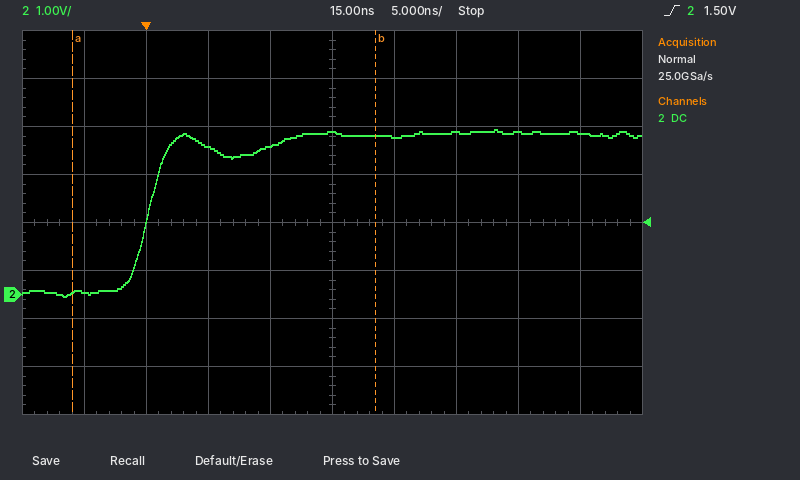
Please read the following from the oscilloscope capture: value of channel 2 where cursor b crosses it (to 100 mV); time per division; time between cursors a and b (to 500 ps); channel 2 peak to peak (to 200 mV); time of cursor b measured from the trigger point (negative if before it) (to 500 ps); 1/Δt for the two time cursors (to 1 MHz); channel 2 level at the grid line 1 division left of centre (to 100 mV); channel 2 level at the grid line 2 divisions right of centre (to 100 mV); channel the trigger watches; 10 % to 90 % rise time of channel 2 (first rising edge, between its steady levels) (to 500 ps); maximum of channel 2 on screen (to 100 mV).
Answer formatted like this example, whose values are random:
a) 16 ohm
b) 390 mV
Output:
a) 3.3 V
b) 5 ns
c) 24.5 ns
d) 3.4 V
e) +18.5 ns
f) 41 MHz
g) 3.1 V
h) 3.4 V
i) channel 2
j) 3.0 ns
k) 3.4 V
